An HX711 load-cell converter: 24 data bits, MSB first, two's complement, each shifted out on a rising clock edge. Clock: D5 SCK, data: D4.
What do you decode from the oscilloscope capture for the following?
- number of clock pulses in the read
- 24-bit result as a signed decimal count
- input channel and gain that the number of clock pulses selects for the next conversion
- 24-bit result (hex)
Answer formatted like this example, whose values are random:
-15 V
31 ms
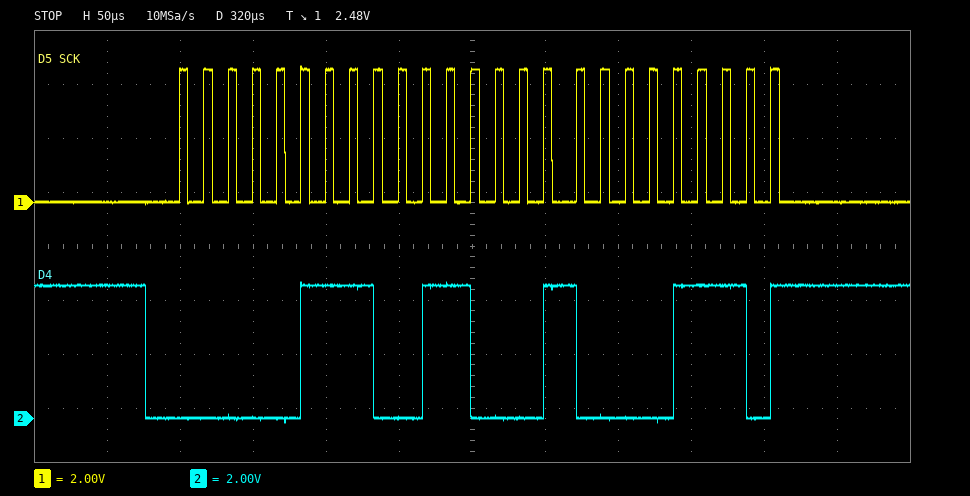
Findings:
25
471310
channel A, gain 128
0x07310E
